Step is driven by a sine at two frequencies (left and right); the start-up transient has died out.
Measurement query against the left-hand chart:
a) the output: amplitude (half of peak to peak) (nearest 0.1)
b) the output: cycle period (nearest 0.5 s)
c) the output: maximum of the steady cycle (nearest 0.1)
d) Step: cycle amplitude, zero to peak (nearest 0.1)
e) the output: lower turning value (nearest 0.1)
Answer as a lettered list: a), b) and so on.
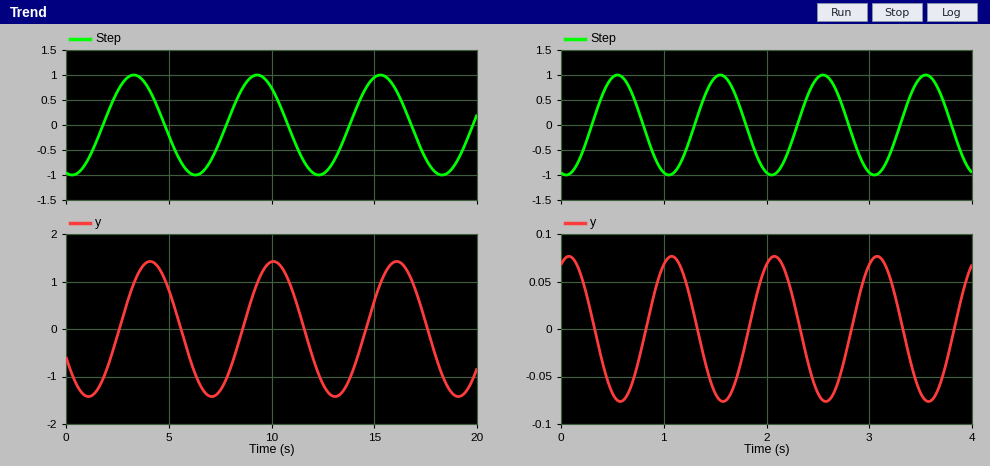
a) 1.4
b) 6.0 s
c) 1.4
d) 1.0
e) -1.4
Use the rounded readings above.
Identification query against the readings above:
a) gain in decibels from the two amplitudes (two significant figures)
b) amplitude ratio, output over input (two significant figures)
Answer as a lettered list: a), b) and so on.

a) 2.9 dB
b) 1.4
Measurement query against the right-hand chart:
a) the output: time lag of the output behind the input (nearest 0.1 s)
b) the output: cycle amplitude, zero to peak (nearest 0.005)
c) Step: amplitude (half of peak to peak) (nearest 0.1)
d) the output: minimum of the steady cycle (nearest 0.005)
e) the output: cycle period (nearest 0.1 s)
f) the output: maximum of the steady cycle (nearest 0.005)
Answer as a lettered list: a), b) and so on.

a) 0.5 s
b) 0.075
c) 1.0
d) -0.075
e) 1.0 s
f) 0.075
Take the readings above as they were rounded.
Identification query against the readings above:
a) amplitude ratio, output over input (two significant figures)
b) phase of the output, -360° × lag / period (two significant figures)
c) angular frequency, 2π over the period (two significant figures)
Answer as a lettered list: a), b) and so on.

a) 0.075
b) -180°
c) 6.3 rad/s
